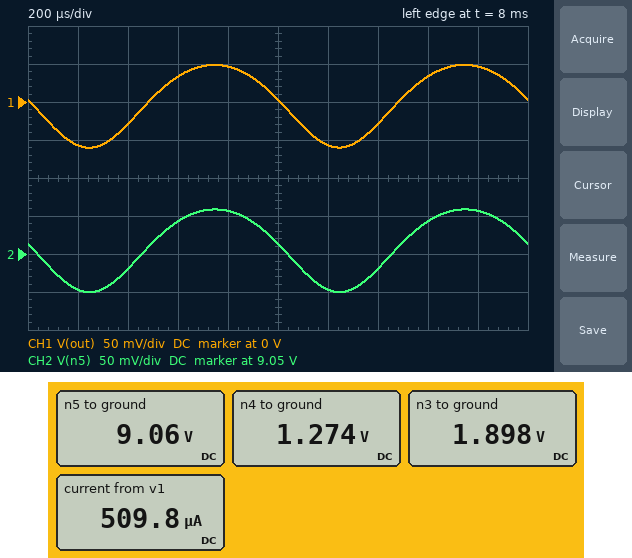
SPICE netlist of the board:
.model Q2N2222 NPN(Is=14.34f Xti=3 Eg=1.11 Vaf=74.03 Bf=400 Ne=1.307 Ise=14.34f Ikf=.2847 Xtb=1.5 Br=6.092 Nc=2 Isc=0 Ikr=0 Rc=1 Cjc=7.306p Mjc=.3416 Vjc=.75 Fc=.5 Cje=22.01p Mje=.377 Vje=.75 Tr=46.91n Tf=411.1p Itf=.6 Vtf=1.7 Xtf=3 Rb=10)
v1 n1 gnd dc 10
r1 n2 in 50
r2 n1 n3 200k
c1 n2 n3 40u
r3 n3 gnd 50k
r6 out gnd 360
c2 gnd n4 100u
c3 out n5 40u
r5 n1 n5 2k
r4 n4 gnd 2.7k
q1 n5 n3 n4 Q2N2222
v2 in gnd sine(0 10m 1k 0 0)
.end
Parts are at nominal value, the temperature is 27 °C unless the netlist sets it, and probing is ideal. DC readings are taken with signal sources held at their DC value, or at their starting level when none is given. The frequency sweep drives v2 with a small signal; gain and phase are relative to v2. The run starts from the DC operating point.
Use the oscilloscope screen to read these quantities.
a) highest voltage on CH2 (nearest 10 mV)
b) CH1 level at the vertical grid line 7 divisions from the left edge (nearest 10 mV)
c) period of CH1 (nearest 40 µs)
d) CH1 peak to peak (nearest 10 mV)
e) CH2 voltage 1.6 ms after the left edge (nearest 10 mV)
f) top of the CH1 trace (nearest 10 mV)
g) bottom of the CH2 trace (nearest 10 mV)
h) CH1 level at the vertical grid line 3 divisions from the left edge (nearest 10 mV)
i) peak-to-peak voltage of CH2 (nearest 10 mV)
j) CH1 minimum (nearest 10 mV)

9.11 V
-30 mV
1.00 ms
110 mV
9.09 V
50 mV
9.00 V
30 mV
110 mV
-60 mV
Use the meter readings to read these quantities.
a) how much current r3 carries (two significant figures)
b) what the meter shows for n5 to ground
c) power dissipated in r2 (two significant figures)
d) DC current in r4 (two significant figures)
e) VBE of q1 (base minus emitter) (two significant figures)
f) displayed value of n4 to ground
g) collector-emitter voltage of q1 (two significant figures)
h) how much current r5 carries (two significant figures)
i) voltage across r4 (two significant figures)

38 µA
9.06 V
330 µW
470 µA
620 mV
1.274 V
7.8 V
470 µA
1.3 V
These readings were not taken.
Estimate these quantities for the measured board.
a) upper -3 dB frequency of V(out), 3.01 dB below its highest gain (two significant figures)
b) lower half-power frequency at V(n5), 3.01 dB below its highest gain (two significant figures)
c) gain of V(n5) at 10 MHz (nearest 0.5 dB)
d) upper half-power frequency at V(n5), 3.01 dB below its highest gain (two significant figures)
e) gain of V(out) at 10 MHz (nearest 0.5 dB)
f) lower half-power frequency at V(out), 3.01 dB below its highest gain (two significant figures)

37 MHz
25 Hz
14.5 dB
37 MHz
14.5 dB
30 Hz
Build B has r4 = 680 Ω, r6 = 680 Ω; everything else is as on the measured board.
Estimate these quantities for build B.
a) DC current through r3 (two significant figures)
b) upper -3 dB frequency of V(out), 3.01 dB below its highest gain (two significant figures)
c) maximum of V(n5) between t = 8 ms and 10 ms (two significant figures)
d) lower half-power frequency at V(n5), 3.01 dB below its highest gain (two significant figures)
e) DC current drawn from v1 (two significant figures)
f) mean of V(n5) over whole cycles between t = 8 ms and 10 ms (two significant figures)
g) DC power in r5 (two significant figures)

34 µA
14 MHz
7.2 V
95 Hz
1.6 mA
6.9 V
4.7 mW
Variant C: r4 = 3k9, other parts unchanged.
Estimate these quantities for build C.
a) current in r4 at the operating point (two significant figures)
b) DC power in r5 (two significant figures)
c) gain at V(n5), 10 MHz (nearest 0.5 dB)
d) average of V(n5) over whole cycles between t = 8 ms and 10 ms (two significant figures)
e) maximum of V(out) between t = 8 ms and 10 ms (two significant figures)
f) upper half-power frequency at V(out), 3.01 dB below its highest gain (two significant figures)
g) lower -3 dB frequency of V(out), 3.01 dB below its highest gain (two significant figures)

340 µA
220 µW
11.5 dB
9.3 V
35 mV
42 MHz
21 Hz
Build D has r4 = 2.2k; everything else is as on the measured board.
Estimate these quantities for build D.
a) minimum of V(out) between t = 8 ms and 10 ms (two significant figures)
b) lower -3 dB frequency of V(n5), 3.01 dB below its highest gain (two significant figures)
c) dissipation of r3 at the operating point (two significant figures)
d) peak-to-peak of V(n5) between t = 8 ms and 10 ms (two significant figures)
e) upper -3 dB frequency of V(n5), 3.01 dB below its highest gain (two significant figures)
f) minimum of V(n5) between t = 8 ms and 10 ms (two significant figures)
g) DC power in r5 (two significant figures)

-72 mV
32 Hz
71 µW
130 mV
34 MHz
8.8 V
640 µW
